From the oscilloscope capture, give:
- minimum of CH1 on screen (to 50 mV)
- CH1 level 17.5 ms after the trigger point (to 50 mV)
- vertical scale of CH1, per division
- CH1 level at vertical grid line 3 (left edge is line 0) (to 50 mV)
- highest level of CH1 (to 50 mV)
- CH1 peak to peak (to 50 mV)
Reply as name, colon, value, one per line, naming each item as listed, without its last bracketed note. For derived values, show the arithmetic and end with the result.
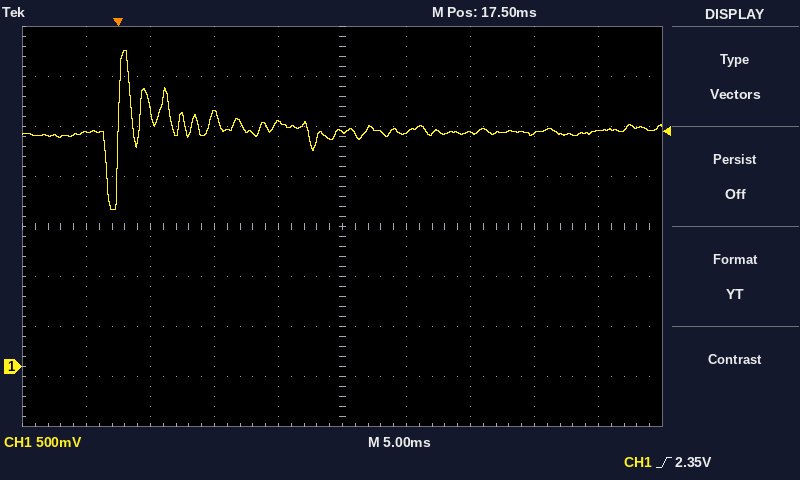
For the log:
minimum of CH1 on screen: 1.55 V
CH1 level 17.5 ms after the trigger point: 2.35 V
vertical scale of CH1, per division: 500 mV
CH1 level at vertical grid line 3 (left edge is line 0): 2.55 V
highest level of CH1: 3.15 V
CH1 peak to peak: 3.15 V − (1.55 V) = 1.60 V
